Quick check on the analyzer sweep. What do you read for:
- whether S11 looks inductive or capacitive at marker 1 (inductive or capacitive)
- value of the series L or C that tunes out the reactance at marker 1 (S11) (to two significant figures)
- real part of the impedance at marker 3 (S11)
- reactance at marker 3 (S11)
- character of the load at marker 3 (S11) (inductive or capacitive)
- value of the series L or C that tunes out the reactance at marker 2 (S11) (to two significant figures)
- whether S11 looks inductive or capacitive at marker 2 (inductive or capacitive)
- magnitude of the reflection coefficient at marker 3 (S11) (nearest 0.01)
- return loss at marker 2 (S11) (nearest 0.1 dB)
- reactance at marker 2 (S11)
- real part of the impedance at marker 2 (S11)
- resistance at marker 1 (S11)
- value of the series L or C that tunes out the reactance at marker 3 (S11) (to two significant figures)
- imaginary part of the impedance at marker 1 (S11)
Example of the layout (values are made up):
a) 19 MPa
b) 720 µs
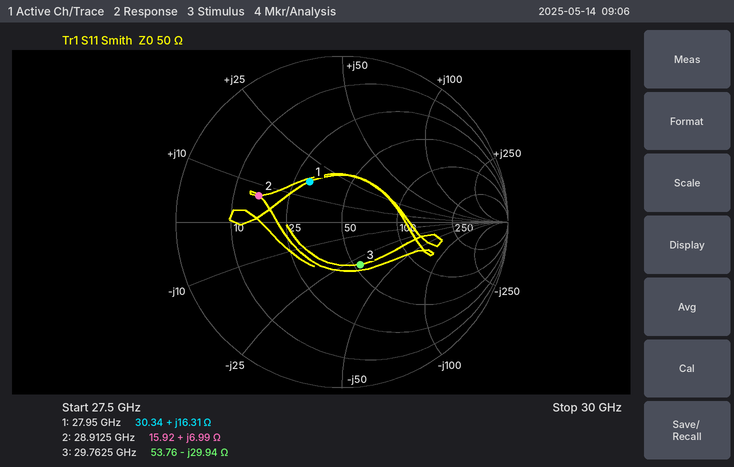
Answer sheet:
a) inductive
b) 350 fF
c) 53.76 Ω
d) -29.94 Ω
e) capacitive
f) 790 fF
g) inductive
h) 0.28
i) 5.6 dB
j) +6.99 Ω
k) 15.92 Ω
l) 30.34 Ω
m) 160 pH
n) +16.31 Ω
